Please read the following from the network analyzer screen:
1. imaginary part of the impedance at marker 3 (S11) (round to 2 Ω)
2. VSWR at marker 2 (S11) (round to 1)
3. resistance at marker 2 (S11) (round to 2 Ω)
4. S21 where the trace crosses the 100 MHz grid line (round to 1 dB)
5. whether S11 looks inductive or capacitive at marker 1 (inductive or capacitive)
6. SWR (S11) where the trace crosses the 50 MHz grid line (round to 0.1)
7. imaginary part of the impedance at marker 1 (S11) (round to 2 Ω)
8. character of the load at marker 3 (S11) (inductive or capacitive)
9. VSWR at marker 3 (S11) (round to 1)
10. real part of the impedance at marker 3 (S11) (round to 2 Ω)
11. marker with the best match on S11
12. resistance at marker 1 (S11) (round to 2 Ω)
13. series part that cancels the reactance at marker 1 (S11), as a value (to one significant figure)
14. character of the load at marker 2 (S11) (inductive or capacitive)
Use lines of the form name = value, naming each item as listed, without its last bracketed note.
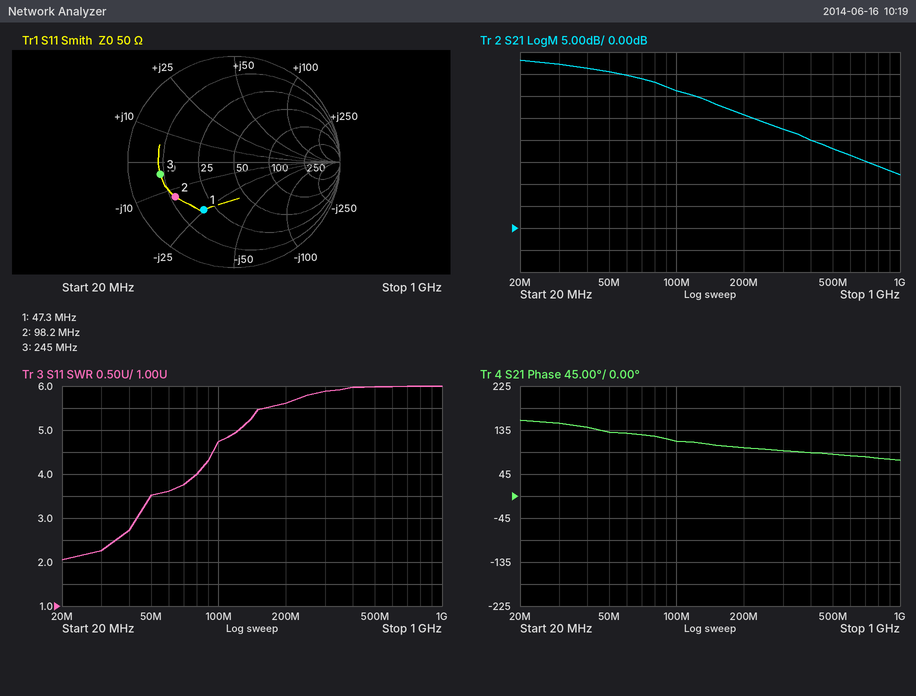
imaginary part of the impedance at marker 3 (S11) = -4 Ω
VSWR at marker 2 (S11) = 5
resistance at marker 2 (S11) = 12 Ω
S21 where the trace crosses the 100 MHz grid line = 31 dB
whether S11 looks inductive or capacitive at marker 1 = capacitive
SWR (S11) where the trace crosses the 50 MHz grid line = 3.5
imaginary part of the impedance at marker 1 (S11) = -24 Ω
character of the load at marker 3 (S11) = capacitive
VSWR at marker 3 (S11) = 6
real part of the impedance at marker 3 (S11) = 8 Ω
marker with the best match on S11 = marker 1
resistance at marker 1 (S11) = 20 Ω
series part that cancels the reactance at marker 1 (S11), as a value = 80 nH
character of the load at marker 2 (S11) = capacitive
